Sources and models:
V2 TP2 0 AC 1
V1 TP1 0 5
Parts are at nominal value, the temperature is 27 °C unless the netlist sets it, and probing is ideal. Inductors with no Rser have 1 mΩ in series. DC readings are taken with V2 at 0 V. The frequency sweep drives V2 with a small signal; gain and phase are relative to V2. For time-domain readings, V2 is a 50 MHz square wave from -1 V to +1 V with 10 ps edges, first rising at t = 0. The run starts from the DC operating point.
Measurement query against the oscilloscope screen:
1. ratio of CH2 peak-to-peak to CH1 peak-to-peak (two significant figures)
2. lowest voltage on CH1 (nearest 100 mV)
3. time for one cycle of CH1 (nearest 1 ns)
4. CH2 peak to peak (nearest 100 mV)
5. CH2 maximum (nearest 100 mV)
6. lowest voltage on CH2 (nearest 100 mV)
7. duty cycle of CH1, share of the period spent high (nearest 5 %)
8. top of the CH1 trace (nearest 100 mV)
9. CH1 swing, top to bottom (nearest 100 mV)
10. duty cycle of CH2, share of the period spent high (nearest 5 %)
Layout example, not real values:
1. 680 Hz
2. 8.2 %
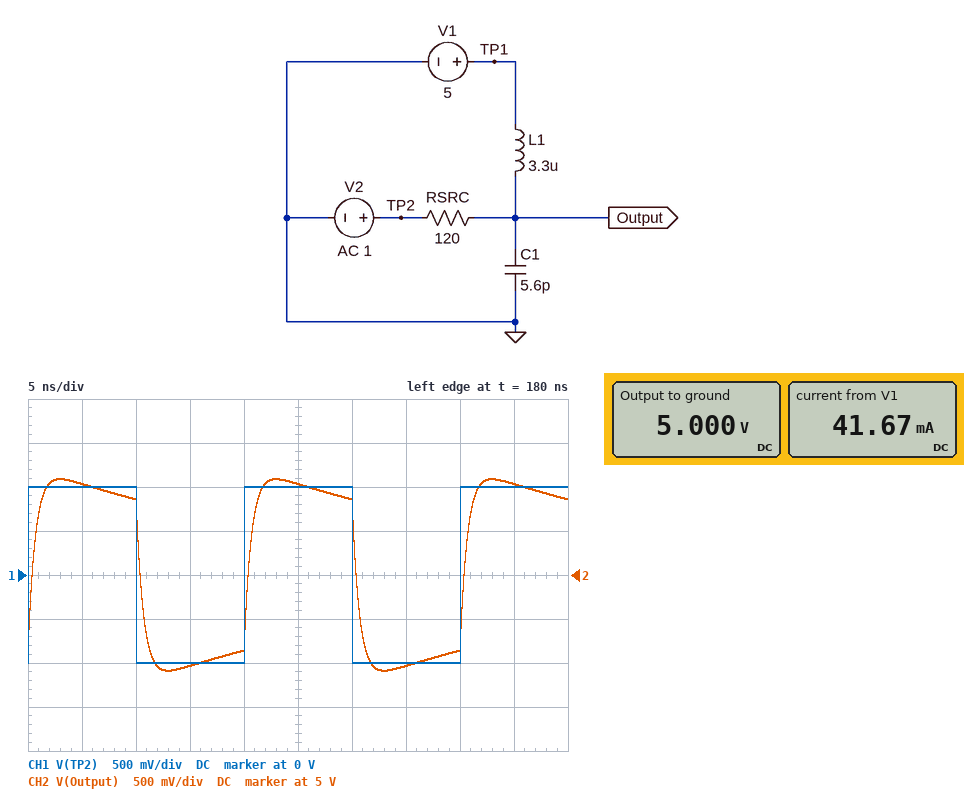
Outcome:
1. 1.1
2. -1.0 V
3. 20 ns
4. 2.2 V
5. 6.1 V
6. 3.9 V
7. 50 %
8. 1.0 V
9. 2.0 V
10. 50 %
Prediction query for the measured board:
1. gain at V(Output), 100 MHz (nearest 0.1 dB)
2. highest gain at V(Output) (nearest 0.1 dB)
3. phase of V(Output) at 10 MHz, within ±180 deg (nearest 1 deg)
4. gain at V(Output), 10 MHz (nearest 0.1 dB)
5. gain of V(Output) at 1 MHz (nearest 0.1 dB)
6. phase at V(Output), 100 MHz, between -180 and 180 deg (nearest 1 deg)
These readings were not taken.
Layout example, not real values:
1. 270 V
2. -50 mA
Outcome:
1. -0.5 dB
2. 0 dB
3. 28 deg
4. -1.1 dB
5. -15.4 dB
6. -20 deg
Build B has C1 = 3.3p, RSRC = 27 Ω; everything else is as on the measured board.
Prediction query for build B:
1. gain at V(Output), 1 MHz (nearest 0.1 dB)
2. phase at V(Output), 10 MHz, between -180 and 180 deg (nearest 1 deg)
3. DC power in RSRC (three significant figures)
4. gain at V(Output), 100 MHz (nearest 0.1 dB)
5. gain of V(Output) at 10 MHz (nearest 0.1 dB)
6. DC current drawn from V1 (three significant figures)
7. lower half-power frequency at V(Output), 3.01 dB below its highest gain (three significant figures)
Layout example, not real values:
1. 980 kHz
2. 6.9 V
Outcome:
1. -4.3 dB
2. 7 deg
3. 926 mW
4. 0 dB
5. -0.1 dB
6. 185 mA
7. 1.30 MHz
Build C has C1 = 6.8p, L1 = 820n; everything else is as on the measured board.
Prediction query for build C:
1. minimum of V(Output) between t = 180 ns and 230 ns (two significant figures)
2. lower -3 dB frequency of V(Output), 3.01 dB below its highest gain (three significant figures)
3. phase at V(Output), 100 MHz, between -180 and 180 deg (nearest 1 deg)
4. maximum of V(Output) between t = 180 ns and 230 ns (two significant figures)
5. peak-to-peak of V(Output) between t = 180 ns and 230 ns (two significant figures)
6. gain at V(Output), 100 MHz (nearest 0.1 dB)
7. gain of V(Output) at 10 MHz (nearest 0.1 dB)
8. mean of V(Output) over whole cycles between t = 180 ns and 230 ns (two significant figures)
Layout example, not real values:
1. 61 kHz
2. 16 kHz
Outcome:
1. 3.7 V
2. 21.0 MHz
3. -16 deg
4. 6.3 V
5. 2.7 V
6. -0.3 dB
7. -7.9 dB
8. 5.0 V
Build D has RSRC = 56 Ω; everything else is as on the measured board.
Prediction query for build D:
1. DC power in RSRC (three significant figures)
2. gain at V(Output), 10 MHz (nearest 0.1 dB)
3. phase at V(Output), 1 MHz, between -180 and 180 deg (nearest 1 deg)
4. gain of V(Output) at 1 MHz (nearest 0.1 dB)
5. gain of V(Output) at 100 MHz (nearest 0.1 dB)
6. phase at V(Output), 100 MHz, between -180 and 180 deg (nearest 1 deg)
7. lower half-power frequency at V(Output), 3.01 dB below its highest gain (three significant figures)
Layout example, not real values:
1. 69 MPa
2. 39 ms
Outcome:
1. 446 mW
2. -0.3 dB
3. 70 deg
4. -9.2 dB
5. -0.1 dB
6. -10 deg
7. 2.69 MHz
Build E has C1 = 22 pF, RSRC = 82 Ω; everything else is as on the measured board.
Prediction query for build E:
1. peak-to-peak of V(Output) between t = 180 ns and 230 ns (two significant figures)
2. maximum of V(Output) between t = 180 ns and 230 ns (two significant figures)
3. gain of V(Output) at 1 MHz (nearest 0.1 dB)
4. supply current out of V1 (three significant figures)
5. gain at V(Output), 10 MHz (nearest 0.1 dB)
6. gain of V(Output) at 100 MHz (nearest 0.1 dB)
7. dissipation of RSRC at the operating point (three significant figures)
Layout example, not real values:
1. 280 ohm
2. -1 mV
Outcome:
1. 2.0 V
2. 6.0 V
3. -12.2 dB
4. 61.0 mA
5. -0.3 dB
6. -3.4 dB
7. 305 mW
